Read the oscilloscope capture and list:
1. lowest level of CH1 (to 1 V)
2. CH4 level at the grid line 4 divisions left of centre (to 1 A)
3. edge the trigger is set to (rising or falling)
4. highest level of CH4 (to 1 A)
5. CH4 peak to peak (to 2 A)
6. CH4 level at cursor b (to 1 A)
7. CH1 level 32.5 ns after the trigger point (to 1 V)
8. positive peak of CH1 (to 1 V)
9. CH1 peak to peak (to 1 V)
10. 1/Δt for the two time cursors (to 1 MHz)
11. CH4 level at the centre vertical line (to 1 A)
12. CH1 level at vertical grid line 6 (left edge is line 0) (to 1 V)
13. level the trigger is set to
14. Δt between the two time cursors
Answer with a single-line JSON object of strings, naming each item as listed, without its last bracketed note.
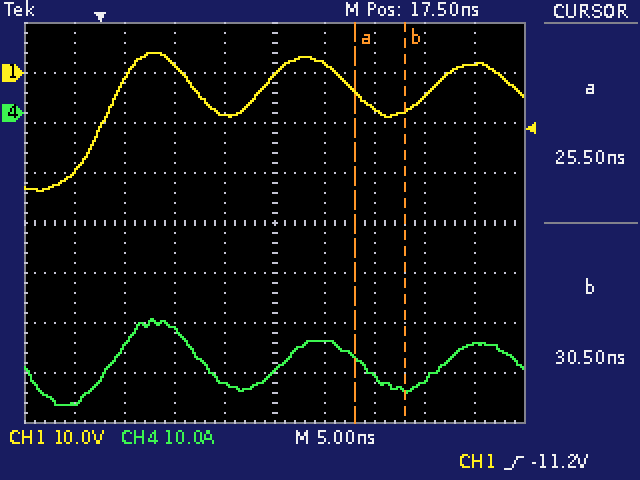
{"lowest level of CH1": "-24 V", "CH4 level at the grid line 4 divisions left of centre": "-58 A", "edge the trigger is set to": "rising", "highest level of CH4": "-41 A", "CH4 peak to peak": "18 A", "CH4 level at cursor b": "-55 A", "CH1 level 32.5 ns after the trigger point": "-5 V", "positive peak of CH1": "4 V", "CH1 peak to peak": "28 V", "1/Δt for the two time cursors": "200 MHz", "CH4 level at the centre vertical line": "-52 A", "CH1 level at vertical grid line 6 (left edge is line 0)": "2 V", "level the trigger is set to": "-11.2 V", "Δt between the two time cursors": "5.0 ns"}
